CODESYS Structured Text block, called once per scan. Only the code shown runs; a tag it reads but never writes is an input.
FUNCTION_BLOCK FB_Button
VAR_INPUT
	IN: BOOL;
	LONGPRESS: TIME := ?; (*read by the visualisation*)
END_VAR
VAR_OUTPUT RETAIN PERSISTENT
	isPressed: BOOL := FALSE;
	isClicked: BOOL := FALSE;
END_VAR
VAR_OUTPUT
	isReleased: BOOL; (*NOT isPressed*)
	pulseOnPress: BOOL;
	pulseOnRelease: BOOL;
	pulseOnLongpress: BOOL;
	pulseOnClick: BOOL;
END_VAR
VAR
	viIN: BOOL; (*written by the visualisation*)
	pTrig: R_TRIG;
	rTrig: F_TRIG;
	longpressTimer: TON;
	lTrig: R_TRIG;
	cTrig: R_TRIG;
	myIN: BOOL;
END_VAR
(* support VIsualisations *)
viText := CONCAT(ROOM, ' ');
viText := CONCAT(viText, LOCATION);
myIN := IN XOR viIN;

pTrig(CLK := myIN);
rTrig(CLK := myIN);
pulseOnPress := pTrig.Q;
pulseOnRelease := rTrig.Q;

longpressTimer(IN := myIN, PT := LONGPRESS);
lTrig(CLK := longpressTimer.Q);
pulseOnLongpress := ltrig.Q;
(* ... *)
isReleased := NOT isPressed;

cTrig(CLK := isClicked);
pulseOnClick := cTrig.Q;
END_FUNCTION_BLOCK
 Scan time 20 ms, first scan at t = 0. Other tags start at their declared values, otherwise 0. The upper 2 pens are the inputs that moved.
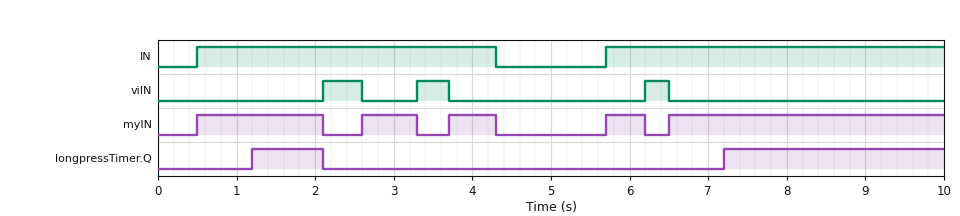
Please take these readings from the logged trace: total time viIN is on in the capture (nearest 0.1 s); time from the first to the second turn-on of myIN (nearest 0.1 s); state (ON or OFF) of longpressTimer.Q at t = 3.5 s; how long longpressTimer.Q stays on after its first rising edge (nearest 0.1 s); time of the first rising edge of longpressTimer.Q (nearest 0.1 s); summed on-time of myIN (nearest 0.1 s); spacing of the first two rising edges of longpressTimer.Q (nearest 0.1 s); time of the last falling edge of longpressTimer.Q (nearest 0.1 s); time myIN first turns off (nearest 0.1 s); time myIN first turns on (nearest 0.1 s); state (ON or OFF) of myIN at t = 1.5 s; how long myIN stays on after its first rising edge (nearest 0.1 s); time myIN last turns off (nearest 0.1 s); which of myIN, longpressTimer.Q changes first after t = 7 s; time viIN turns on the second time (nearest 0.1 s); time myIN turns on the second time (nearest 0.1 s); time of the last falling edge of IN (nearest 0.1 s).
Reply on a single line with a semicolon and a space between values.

1.2 s; 2.1 s; OFF; 0.9 s; 1.2 s; 6.9 s; 6.0 s; 2.1 s; 2.1 s; 0.5 s; ON; 1.6 s; 6.2 s; longpressTimer.Q; 3.3 s; 2.6 s; 4.3 s
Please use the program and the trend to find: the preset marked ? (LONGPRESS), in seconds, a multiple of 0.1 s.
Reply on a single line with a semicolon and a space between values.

0.7 s
